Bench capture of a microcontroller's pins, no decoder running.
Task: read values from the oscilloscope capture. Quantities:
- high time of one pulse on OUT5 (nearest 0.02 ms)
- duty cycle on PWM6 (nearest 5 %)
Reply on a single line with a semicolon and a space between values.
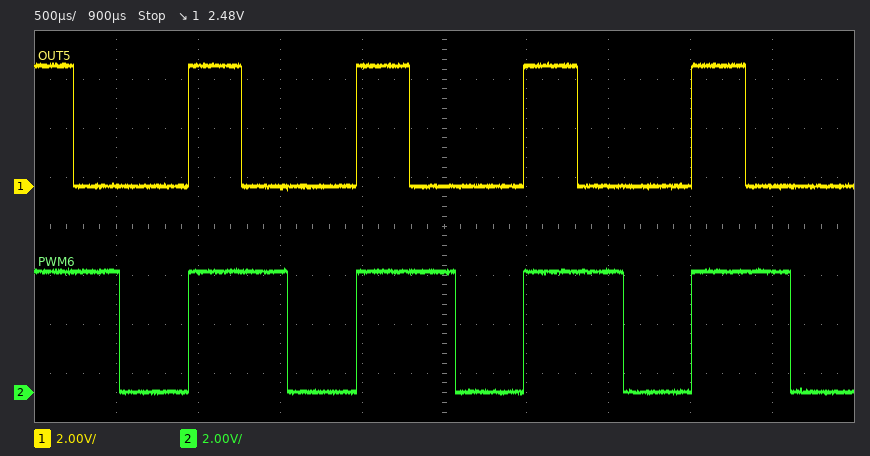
0.32 ms; 60 %
